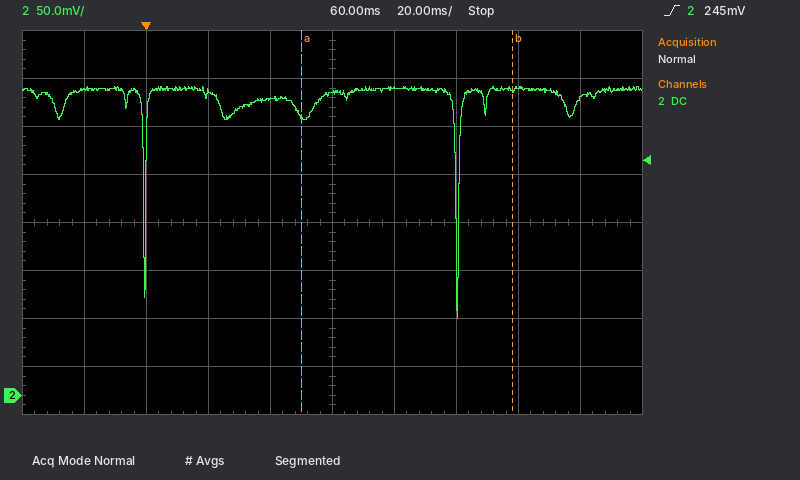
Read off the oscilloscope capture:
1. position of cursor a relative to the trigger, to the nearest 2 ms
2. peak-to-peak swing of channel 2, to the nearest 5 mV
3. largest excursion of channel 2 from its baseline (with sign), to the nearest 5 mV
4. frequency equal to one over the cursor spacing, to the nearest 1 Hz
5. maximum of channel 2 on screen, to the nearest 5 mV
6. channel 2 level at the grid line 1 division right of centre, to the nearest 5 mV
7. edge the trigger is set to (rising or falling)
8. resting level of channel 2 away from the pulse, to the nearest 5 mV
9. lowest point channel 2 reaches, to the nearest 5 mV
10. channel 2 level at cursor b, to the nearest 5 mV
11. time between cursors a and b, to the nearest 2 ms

+50 ms
240 mV
-240 mV
15 Hz
320 mV
320 mV
rising
320 mV
80 mV
320 mV
68 ms
